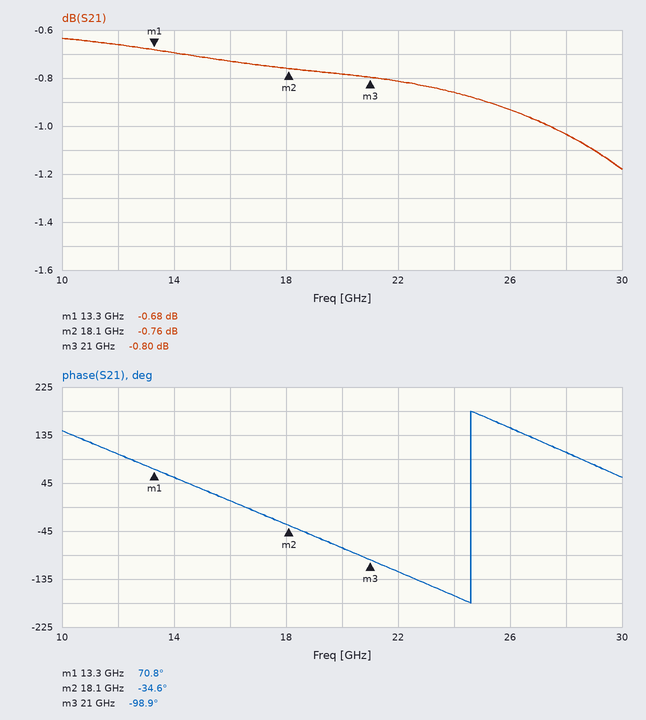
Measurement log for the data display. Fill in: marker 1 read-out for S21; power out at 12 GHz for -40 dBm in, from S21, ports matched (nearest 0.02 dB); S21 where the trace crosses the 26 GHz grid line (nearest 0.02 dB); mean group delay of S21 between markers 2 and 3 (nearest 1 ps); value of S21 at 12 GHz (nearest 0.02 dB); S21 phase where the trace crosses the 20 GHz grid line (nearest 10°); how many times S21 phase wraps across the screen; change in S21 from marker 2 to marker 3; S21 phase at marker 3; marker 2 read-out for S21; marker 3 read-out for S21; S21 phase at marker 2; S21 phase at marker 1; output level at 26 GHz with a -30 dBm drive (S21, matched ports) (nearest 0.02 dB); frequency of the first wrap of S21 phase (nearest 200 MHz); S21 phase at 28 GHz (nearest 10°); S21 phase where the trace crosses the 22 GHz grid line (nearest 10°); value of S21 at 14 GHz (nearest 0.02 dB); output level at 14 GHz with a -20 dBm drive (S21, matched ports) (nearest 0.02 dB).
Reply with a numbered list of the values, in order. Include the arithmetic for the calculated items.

1. -0.68 dB
2. -40 dBm + (-0.66 dB) = -40.66 dBm
3. -0.94 dB
4. −(-98.9° − (-34.6°))/(360° × 2.9 GHz) ≈ 62 ps
5. -0.66 dB
6. -80°
7. 1
8. -0.8 − (-0.76) = -0.04 dB
9. -98.9°
10. -0.76 dB
11. -0.80 dB
12. -34.6°
13. 70.8°
14. -30 dBm + (-0.94 dB) = -30.94 dBm
15. 24.6 GHz
16. 100°
17. -120°
18. -0.70 dB
19. -20 dBm + (-0.70 dB) = -20.70 dBm
